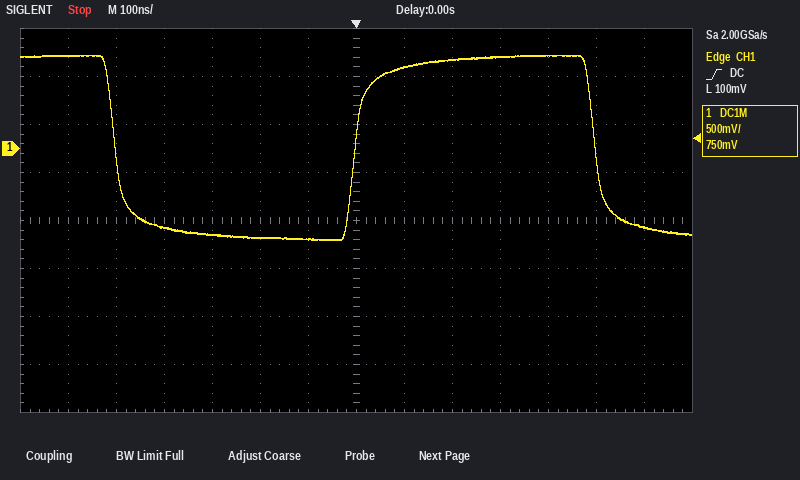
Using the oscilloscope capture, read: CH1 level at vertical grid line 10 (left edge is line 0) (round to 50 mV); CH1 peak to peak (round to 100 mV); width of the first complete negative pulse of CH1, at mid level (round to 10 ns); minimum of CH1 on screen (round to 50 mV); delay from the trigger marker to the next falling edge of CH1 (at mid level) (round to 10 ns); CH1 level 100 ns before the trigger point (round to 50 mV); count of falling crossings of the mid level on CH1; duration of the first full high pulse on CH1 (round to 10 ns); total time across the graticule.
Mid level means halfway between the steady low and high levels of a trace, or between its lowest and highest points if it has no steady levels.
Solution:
950 mV
1.90 V
500 ns
-950 mV
500 ns
-950 mV
2
500 ns
1.4 µs
